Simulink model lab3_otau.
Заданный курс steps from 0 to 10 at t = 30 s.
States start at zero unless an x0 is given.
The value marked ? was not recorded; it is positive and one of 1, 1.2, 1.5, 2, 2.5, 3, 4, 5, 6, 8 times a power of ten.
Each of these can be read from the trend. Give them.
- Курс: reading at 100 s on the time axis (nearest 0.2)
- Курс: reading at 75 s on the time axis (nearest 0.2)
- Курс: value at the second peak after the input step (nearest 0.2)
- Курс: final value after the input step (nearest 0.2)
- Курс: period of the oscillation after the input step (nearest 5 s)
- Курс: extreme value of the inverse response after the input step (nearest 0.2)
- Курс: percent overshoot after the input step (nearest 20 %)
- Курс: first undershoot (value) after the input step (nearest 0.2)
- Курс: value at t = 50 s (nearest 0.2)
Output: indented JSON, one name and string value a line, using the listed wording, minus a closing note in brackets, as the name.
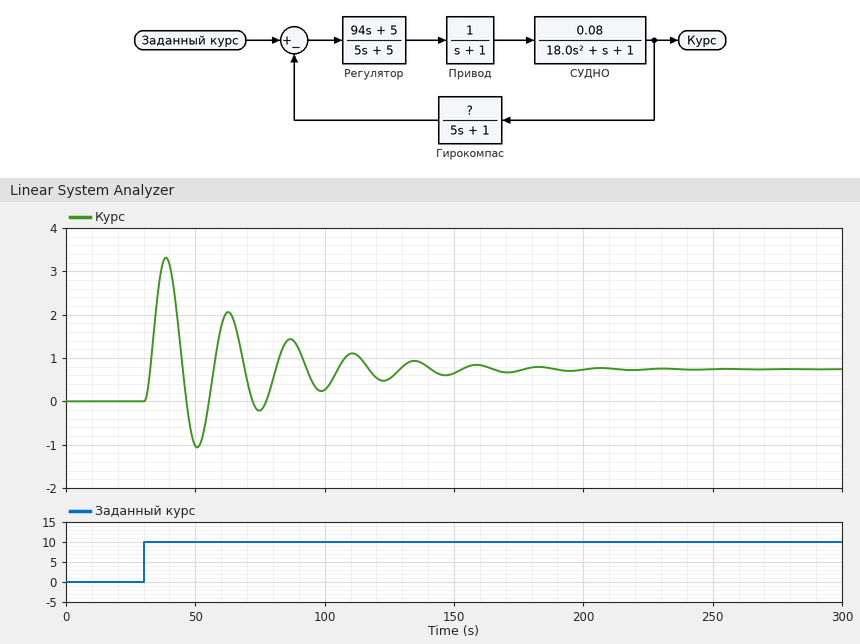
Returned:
{
  "Курс: reading at 100 s on the time axis": "0.2",
  "Курс: reading at 75 s on the time axis": "-0.2",
  "Курс: value at the second peak after the input step": "2.0",
  "Курс: final value after the input step": "0.8",
  "Курс: period of the oscillation after the input step": "25 s",
  "Курс: extreme value of the inverse response after the input step": "-1.0",
  "Курс: percent overshoot after the input step": "340 %",
  "Курс: first undershoot (value) after the input step": "-1.0",
  "Курс: value at t = 50 s": "-1.0"
}
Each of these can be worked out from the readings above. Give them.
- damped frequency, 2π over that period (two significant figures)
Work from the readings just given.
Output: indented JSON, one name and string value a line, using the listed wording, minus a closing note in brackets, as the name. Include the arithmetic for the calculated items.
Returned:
{
  "damped frequency, 2π over that period": "2π / 25 = 0.25 rad/s"
}
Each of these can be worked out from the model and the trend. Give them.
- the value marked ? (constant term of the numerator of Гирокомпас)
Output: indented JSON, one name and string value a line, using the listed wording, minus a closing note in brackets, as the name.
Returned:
{
  "the value marked ?": "1"
}
